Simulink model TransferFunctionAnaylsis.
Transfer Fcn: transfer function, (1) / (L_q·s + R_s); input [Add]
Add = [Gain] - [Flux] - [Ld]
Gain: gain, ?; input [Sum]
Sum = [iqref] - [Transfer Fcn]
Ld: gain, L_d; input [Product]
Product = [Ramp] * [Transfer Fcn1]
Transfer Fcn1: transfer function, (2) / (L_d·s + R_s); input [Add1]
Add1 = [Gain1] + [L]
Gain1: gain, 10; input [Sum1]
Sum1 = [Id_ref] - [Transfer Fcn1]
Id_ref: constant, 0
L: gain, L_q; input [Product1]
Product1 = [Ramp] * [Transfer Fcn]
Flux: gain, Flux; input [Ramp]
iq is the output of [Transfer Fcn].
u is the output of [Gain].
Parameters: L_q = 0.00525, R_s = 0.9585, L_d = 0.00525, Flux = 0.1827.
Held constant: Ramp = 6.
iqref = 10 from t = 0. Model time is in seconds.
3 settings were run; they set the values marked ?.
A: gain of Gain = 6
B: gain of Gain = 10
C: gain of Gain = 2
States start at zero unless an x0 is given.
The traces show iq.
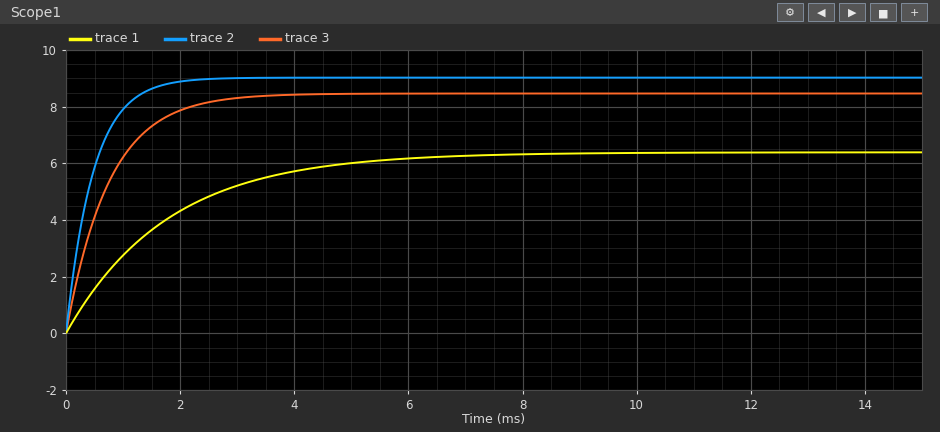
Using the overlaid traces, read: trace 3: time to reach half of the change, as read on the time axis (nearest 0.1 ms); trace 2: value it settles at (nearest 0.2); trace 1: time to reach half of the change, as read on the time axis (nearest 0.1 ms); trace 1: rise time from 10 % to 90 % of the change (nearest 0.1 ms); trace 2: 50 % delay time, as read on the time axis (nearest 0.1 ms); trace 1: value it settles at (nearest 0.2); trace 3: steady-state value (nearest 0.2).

0.5 ms
9.0
1.2 ms
3.9 ms
0.3 ms
6.4
8.4
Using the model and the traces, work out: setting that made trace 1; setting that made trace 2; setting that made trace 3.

C
B
A
